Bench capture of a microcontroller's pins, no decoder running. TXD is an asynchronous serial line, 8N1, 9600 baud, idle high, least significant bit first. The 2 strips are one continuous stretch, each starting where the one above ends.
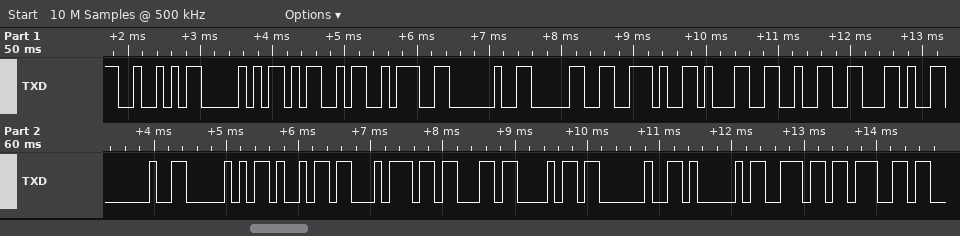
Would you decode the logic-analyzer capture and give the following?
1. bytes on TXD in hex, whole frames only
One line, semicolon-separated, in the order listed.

0x52 0x50 0x4D 0x3A 0x20 0x30 0x2E 0x31 0x32 0x2C 0x20 0x50 0x69 0x74 0x63 0x68 0x20 0x41 0x6E 0x67
